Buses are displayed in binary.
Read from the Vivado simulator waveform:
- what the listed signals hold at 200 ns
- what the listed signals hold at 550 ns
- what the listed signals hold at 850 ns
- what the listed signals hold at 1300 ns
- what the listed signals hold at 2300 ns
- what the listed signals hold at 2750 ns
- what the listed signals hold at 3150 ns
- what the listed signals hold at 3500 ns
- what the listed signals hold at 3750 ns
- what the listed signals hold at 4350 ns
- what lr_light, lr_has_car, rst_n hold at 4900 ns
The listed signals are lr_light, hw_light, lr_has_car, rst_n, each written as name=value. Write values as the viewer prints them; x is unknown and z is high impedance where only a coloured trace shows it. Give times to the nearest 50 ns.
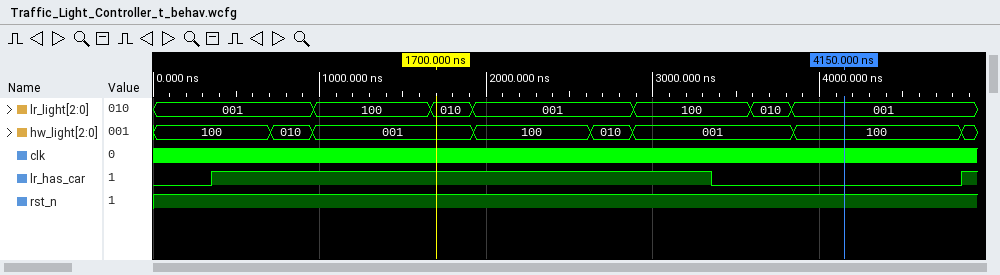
lr_light=001, hw_light=100, lr_has_car=0, rst_n=1
lr_light=001, hw_light=100, lr_has_car=1, rst_n=1
lr_light=001, hw_light=010, lr_has_car=1, rst_n=1
lr_light=100, hw_light=001, lr_has_car=1, rst_n=1
lr_light=001, hw_light=100, lr_has_car=1, rst_n=1
lr_light=001, hw_light=010, lr_has_car=1, rst_n=1
lr_light=100, hw_light=001, lr_has_car=1, rst_n=1
lr_light=100, hw_light=001, lr_has_car=0, rst_n=1
lr_light=010, hw_light=001, lr_has_car=0, rst_n=1
lr_light=001, hw_light=100, lr_has_car=0, rst_n=1
lr_light=001, lr_has_car=1, rst_n=1
